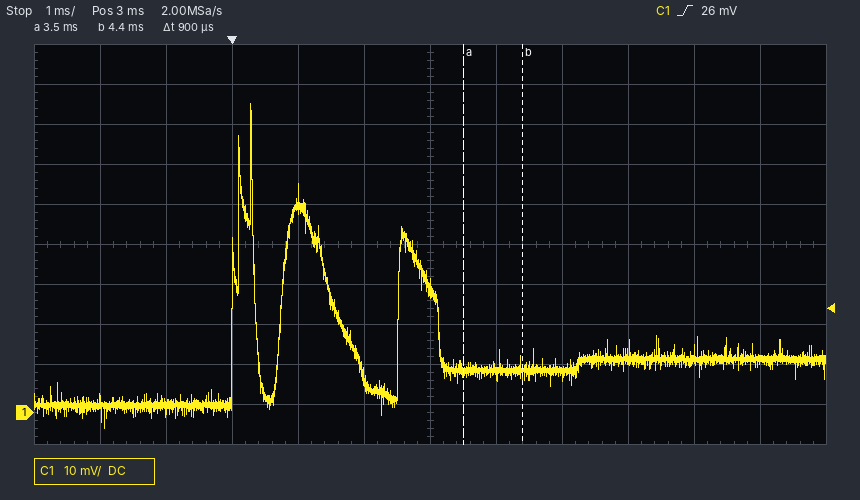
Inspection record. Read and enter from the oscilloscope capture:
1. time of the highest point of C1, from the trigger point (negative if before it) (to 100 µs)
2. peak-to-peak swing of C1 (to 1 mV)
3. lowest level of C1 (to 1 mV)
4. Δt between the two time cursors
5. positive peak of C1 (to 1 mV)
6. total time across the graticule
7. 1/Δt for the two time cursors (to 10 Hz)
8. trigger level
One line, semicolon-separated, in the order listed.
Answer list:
+300 µs; 81 mV; -4 mV; 900 µs; 77 mV; 12 ms; 1.11 kHz; 26 mV
